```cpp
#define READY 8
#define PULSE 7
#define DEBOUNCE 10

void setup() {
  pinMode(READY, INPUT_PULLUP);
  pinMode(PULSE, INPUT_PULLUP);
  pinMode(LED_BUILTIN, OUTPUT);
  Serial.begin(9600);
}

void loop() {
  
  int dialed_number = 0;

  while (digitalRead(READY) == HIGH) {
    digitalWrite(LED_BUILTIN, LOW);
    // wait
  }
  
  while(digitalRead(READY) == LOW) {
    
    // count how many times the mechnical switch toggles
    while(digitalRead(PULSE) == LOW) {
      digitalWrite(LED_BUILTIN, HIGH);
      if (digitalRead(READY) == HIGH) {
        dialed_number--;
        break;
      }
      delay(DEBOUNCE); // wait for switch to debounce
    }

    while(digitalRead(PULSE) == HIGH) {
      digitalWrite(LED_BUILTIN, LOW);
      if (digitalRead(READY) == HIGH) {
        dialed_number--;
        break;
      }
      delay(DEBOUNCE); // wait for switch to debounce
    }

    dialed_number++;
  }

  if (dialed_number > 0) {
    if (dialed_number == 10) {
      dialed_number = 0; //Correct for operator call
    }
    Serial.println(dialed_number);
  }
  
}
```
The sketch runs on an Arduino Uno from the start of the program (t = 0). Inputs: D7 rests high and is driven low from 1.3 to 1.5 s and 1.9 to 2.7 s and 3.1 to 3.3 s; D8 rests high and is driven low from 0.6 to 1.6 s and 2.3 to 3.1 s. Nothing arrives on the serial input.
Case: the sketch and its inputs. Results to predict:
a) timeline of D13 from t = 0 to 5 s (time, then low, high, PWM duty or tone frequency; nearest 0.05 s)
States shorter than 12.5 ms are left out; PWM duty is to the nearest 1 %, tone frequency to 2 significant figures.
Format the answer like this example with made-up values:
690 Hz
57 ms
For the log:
0 s low; 1.3 s high; 1.5 s low; 2.3 s high; 2.7 s low
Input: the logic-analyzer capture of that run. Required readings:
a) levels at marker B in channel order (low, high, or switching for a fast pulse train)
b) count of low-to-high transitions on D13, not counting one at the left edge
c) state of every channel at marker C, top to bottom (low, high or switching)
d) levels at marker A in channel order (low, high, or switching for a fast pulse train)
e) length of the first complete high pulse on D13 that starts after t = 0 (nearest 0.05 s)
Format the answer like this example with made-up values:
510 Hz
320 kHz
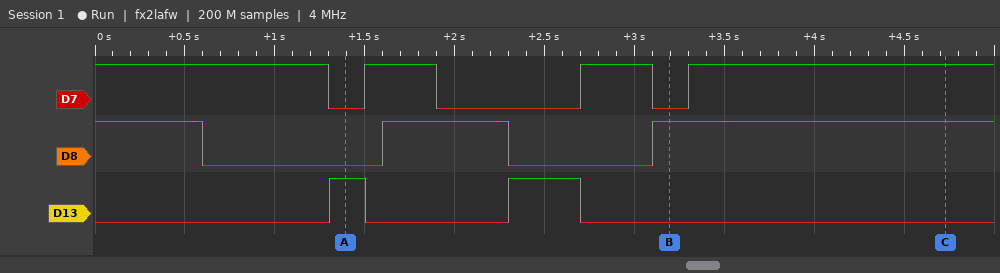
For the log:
D7 low, D8 high, D13 low
2
D7 high, D8 high, D13 low
D7 low, D8 low, D13 high
0.20 s
